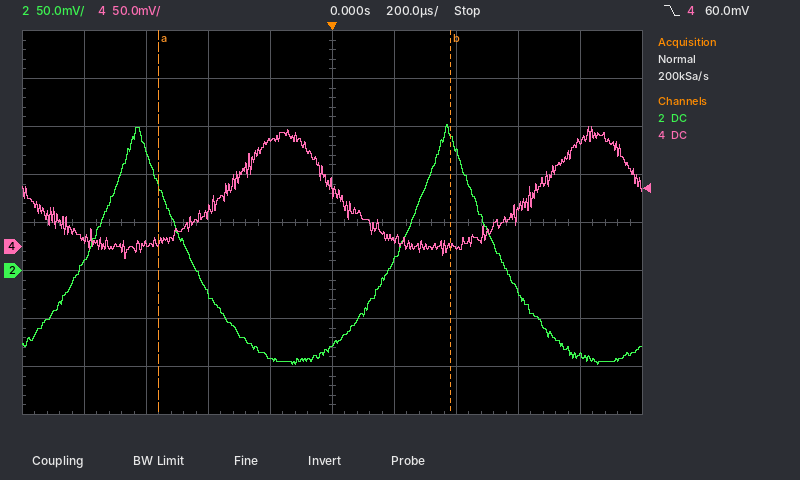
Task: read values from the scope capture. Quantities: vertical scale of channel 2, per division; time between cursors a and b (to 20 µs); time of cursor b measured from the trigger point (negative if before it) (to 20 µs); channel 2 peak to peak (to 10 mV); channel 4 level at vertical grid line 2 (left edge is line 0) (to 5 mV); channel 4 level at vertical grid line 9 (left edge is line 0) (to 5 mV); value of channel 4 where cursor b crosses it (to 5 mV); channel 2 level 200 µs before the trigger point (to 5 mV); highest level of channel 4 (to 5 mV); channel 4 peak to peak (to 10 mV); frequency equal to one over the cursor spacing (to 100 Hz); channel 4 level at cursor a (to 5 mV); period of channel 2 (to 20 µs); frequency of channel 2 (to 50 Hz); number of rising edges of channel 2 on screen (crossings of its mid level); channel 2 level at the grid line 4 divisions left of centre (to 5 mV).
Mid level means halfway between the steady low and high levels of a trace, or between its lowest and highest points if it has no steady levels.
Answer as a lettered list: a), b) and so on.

a) 50 mV
b) 940 µs
c) +380 µs
d) 250 mV
e) 5 mV
f) 110 mV
g) 0 mV
h) -90 mV
i) 125 mV
j) 140 mV
k) 1.1 kHz
l) 5 mV
m) 1.00 ms
n) 1.00 kHz
o) 2
p) 10 mV
